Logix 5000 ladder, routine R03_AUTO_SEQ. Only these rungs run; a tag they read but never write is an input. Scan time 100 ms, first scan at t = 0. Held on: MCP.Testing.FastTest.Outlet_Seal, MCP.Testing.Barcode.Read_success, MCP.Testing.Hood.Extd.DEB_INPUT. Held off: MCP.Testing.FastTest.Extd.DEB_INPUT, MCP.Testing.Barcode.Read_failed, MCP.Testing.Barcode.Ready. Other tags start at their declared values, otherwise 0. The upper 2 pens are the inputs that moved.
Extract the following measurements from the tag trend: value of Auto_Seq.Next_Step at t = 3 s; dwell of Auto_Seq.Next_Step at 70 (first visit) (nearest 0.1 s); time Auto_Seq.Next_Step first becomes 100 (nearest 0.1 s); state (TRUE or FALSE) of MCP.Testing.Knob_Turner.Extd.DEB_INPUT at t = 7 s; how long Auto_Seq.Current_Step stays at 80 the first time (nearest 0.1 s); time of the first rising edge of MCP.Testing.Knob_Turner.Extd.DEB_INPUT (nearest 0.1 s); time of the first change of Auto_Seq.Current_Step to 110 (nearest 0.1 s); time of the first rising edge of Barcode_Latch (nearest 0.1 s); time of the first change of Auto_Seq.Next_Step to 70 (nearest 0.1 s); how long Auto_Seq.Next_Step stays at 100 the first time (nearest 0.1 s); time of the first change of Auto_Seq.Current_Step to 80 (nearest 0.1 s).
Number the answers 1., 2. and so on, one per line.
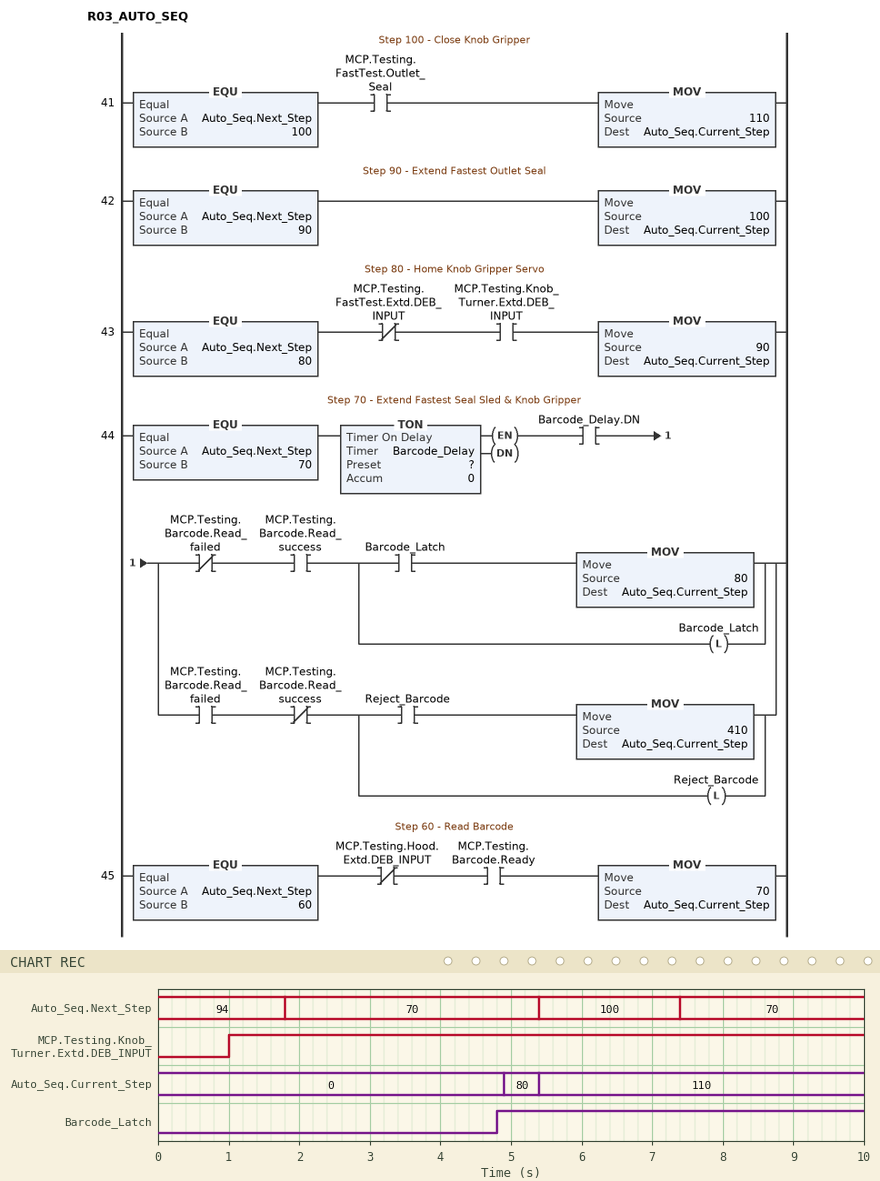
1. 70
2. 3.6 s
3. 5.4 s
4. TRUE
5. 0.5 s
6. 1.0 s
7. 5.4 s
8. 4.8 s
9. 1.8 s
10. 2.0 s
11. 4.9 s
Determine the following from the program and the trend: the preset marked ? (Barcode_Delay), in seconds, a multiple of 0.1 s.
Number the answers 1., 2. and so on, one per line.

1. 3.0 s
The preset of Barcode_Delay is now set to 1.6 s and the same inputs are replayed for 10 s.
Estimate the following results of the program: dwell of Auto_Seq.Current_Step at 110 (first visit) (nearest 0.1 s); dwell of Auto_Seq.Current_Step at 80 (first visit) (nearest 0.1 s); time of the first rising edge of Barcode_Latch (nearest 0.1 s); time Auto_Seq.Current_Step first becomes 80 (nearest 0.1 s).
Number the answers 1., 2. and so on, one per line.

1. 3.6 s
2. 1.9 s
3. 3.4 s
4. 3.5 s
